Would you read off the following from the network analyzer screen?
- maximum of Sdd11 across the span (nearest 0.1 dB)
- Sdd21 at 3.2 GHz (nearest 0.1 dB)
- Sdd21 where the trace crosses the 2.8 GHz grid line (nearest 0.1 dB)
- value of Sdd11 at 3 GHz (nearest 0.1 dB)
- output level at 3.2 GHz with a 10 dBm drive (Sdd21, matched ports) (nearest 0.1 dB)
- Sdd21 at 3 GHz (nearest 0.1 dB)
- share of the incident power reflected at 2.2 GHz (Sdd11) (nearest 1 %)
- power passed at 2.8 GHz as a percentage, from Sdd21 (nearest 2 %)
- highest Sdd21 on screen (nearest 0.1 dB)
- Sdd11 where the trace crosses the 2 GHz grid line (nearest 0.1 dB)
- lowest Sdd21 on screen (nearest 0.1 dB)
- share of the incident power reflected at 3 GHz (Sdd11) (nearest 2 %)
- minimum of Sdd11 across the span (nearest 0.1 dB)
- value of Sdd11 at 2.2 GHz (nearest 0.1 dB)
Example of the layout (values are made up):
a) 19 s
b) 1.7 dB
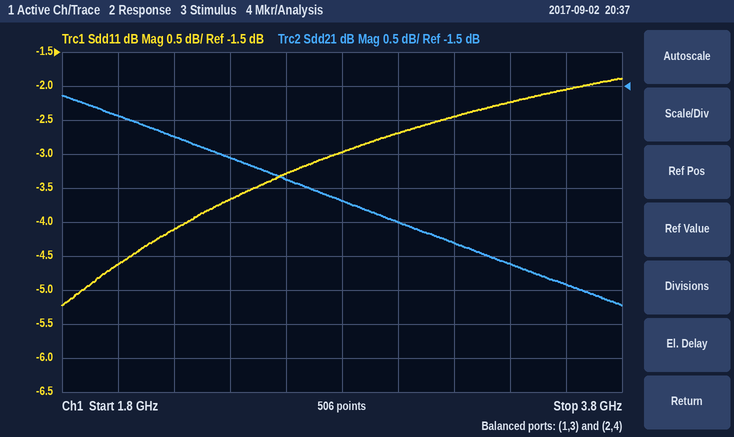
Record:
a) -1.9 dB
b) -3.8 dB
c) -3.2 dB
d) -2.7 dB
e) 6.2 dBm
f) -3.5 dB
g) 39 %
h) 48 %
i) -1.6 dB
j) -4.6 dB
k) -4.7 dB
l) 54 %
m) -5.2 dB
n) -4.1 dB
